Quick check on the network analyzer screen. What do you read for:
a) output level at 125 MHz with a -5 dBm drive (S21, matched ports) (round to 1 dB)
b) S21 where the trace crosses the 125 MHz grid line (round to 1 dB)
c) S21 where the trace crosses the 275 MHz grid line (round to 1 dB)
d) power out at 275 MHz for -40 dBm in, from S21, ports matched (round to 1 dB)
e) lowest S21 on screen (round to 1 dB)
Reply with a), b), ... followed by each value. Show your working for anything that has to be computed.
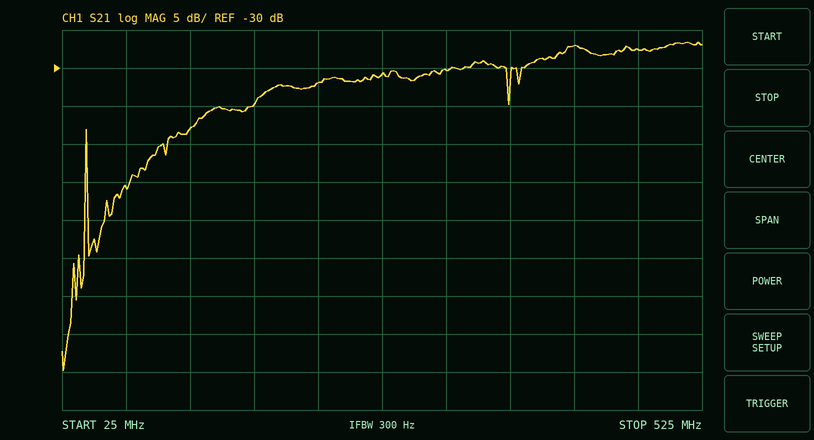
a) -5 dBm + (-38 dB) = -43 dBm
b) -38 dB
c) -31 dB
d) -40 dBm + (-31 dB) = -71 dBm
e) -70 dB
